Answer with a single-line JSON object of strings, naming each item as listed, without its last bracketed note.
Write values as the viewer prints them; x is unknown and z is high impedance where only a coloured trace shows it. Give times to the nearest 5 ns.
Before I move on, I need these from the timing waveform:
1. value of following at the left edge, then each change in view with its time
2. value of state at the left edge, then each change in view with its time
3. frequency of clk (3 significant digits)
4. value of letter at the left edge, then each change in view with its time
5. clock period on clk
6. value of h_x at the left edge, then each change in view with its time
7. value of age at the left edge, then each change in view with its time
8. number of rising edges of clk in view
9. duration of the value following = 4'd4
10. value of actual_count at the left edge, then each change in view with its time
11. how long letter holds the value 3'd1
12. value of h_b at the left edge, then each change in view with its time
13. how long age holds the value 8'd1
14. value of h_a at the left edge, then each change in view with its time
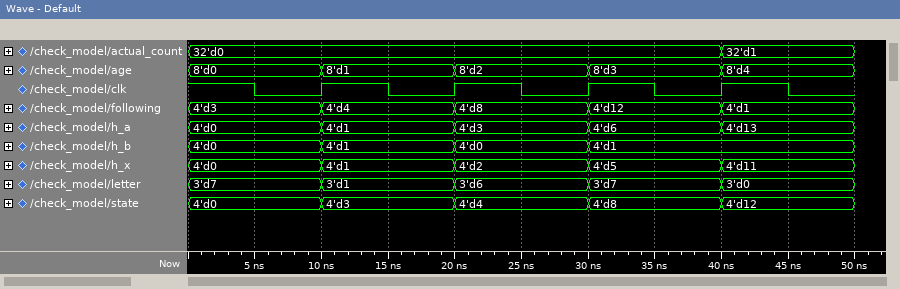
{"value of following at the left edge, then each change in view with its time": "4'd3, 4'd4 at 10 ns, 4'd8 at 20 ns, 4'd12 at 30 ns, 4'd1 at 40 ns", "value of state at the left edge, then each change in view with its time": "4'd0, 4'd3 at 10 ns, 4'd4 at 20 ns, 4'd8 at 30 ns, 4'd12 at 40 ns", "frequency of clk": "100 MHz", "value of letter at the left edge, then each change in view with its time": "3'd7, 3'd1 at 10 ns, 3'd6 at 20 ns, 3'd7 at 30 ns, 3'd0 at 40 ns", "clock period on clk": "10 ns", "value of h_x at the left edge, then each change in view with its time": "4'd0, 4'd1 at 10 ns, 4'd2 at 20 ns, 4'd5 at 30 ns, 4'd11 at 40 ns", "value of age at the left edge, then each change in view with its time": "8'd0, 8'd1 at 10 ns, 8'd2 at 20 ns, 8'd3 at 30 ns, 8'd4 at 40 ns", "number of rising edges of clk in view": "4", "duration of the value following = 4'd4": "10 ns", "value of actual_count at the left edge, then each change in view with its time": "32'd0, 32'd1 at 40 ns", "how long letter holds the value 3'd1": "10 ns", "value of h_b at the left edge, then each change in view with its time": "4'd0, 4'd1 at 10 ns, 4'd0 at 20 ns, 4'd1 at 30 ns", "how long age holds the value 8'd1": "10 ns", "value of h_a at the left edge, then each change in view with its time": "4'd0, 4'd1 at 10 ns, 4'd3 at 20 ns, 4'd6 at 30 ns, 4'd13 at 40 ns"}
